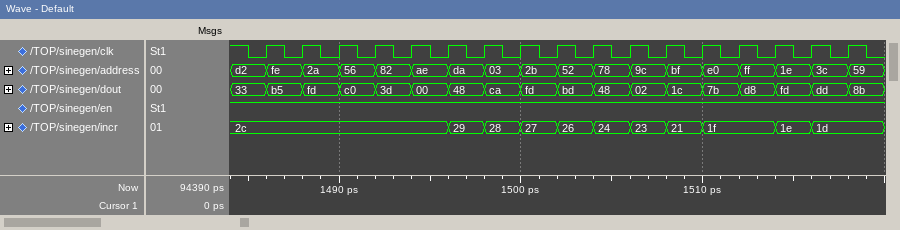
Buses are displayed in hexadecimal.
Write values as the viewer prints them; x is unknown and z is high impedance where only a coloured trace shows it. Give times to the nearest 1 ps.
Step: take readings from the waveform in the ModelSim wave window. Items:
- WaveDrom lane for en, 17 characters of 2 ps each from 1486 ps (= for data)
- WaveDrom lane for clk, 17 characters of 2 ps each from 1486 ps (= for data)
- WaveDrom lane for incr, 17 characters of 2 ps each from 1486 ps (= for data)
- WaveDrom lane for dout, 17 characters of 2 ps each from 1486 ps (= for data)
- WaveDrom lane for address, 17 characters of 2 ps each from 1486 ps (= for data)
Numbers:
{name: 'en', wave: '1................'}
{name: 'clk', wave: 'p................'}
{name: 'incr', wave: '=....========.==.', data: '2c 29 28 27 26 24 23 21 1f 1e 1d'}
{name: 'dout', wave: '=================', data: 'b5 fd c0 3d 00 48 ca fd bd 48 02 1c 7b d8 fd dd 8b'}
{name: 'address', wave: '=================', data: 'fe 2a 56 82 ae da 03 2b 52 78 9c bf e0 ff 1e 3c 59'}
